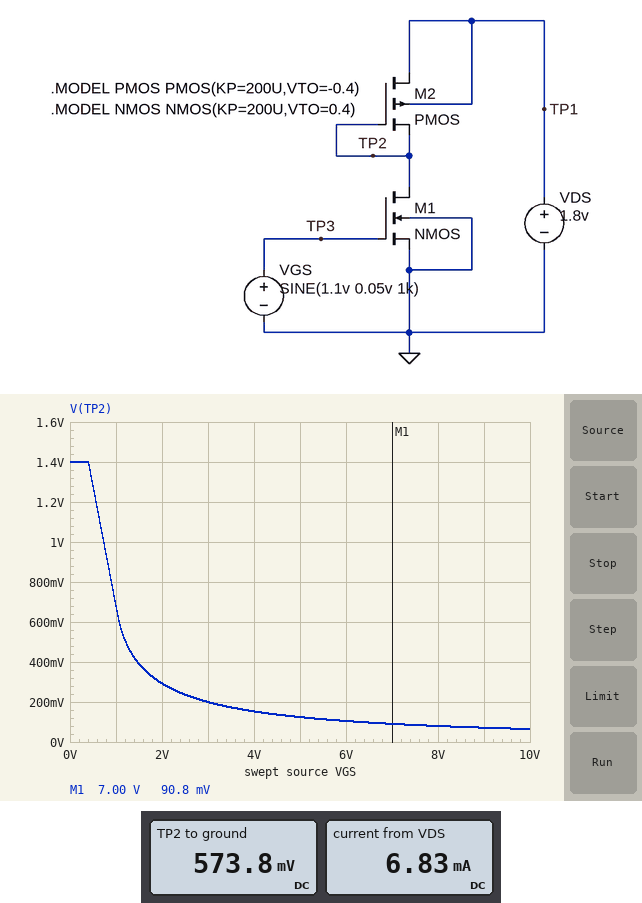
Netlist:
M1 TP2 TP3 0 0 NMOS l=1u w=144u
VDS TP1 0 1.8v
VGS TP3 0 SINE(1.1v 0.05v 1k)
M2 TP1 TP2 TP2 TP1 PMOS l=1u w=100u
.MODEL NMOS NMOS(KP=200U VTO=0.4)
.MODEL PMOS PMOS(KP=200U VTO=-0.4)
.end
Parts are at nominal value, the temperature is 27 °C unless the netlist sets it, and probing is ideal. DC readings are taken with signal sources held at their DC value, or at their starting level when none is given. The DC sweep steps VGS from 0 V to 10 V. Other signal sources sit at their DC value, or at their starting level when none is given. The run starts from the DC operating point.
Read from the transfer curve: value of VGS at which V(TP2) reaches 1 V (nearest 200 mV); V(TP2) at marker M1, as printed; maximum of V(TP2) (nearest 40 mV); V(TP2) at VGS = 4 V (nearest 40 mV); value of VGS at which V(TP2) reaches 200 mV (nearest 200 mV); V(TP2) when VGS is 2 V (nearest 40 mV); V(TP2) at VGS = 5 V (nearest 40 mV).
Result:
800 mV
90.8 mV
1.40 V
160 mV
3.0 V
280 mV
120 mV
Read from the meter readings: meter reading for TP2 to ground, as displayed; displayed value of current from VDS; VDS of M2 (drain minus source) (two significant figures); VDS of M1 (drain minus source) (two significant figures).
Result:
573.8 mV
6.83 mA
1.2 V
570 mV
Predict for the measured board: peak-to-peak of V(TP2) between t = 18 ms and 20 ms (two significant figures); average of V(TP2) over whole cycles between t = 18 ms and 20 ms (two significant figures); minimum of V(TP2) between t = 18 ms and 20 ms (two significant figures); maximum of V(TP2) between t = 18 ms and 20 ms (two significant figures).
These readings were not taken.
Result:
84 mV
580 mV
540 mV
620 mV
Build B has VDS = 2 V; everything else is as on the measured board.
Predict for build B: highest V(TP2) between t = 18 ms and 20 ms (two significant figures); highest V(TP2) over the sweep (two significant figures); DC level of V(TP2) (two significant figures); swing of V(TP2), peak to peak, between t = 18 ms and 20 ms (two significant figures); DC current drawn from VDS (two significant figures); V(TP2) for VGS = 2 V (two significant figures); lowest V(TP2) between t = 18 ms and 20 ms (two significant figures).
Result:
820 mV
1.6 V
760 mV
120 mV
7.1 mA
370 mV
700 mV
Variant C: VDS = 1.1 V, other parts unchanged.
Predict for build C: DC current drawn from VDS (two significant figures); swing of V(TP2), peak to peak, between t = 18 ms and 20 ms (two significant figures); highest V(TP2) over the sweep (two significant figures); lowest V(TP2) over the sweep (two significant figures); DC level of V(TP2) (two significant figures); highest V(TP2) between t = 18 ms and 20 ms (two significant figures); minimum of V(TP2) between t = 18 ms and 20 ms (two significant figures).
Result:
2.9 mA
18 mV
700 mV
17 mV
160 mV
170 mV
150 mV
